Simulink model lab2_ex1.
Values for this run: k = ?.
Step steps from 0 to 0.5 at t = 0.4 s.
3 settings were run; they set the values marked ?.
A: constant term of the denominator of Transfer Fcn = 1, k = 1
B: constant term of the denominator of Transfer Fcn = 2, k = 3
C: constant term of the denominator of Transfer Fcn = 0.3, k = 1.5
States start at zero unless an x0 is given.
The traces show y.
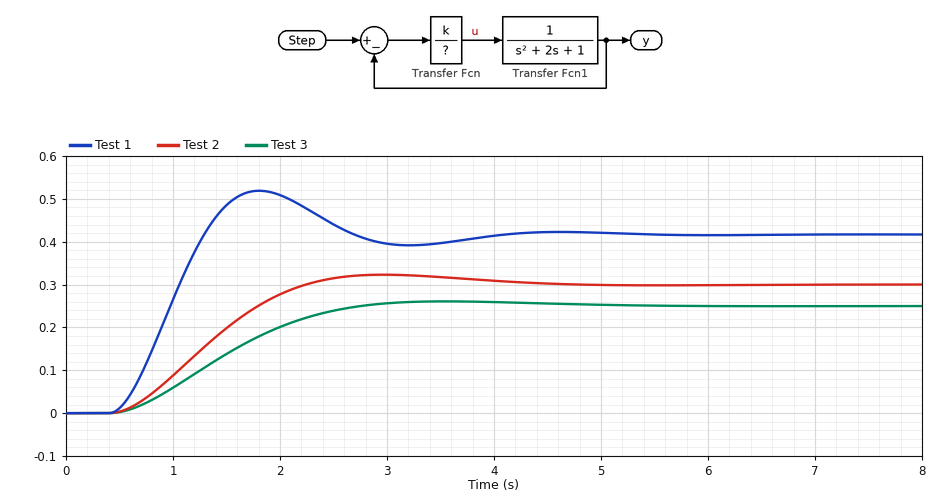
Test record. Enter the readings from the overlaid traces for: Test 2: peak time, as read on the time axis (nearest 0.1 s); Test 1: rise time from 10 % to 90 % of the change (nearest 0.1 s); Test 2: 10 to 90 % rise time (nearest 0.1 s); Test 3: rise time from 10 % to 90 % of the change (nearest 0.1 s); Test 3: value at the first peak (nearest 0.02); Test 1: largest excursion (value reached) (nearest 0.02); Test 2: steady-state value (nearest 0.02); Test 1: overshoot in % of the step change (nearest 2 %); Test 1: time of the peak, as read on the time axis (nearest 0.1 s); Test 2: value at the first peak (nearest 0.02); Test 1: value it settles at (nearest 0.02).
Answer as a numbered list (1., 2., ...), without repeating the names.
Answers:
1. 3.0 s
2. 0.6 s
3. 1.2 s
4. 1.5 s
5. 0.26
6. 0.52
7. 0.30
8. 24 %
9. 1.8 s
10. 0.32
11. 0.42
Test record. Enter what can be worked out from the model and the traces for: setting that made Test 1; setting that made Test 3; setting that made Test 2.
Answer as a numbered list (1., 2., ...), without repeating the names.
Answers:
1. C
2. A
3. B
